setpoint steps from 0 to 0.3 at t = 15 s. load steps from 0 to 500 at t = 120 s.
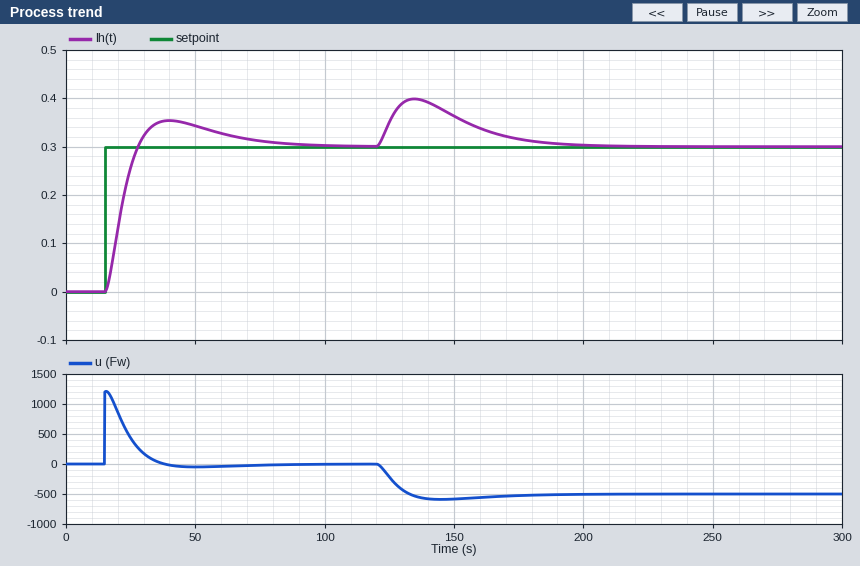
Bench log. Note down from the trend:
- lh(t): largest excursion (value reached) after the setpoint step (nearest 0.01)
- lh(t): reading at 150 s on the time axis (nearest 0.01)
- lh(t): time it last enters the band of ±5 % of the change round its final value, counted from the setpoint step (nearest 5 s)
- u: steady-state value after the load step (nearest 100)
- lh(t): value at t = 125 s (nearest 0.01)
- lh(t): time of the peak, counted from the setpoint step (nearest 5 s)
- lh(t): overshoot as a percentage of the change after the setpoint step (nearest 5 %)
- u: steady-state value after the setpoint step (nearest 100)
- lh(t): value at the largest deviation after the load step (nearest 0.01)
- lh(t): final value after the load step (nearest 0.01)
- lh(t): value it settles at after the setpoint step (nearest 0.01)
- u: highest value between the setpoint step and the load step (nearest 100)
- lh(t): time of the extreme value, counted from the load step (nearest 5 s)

0.35
0.36
55 s
-500
0.35
25 s
20 %
0
0.40
0.30
0.30
1200
15 s
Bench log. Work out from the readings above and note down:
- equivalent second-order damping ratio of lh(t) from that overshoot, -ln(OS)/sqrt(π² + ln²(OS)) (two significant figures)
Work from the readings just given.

0.46
